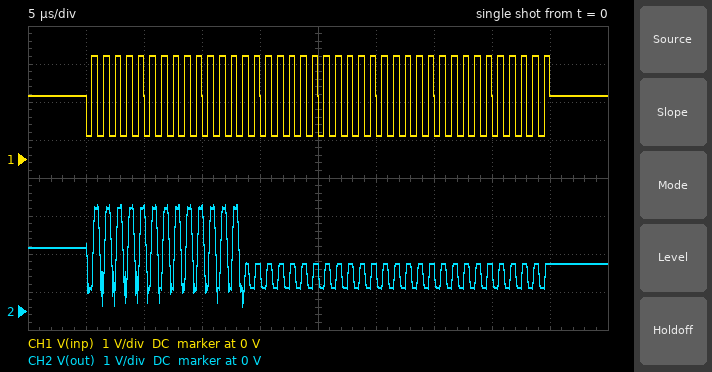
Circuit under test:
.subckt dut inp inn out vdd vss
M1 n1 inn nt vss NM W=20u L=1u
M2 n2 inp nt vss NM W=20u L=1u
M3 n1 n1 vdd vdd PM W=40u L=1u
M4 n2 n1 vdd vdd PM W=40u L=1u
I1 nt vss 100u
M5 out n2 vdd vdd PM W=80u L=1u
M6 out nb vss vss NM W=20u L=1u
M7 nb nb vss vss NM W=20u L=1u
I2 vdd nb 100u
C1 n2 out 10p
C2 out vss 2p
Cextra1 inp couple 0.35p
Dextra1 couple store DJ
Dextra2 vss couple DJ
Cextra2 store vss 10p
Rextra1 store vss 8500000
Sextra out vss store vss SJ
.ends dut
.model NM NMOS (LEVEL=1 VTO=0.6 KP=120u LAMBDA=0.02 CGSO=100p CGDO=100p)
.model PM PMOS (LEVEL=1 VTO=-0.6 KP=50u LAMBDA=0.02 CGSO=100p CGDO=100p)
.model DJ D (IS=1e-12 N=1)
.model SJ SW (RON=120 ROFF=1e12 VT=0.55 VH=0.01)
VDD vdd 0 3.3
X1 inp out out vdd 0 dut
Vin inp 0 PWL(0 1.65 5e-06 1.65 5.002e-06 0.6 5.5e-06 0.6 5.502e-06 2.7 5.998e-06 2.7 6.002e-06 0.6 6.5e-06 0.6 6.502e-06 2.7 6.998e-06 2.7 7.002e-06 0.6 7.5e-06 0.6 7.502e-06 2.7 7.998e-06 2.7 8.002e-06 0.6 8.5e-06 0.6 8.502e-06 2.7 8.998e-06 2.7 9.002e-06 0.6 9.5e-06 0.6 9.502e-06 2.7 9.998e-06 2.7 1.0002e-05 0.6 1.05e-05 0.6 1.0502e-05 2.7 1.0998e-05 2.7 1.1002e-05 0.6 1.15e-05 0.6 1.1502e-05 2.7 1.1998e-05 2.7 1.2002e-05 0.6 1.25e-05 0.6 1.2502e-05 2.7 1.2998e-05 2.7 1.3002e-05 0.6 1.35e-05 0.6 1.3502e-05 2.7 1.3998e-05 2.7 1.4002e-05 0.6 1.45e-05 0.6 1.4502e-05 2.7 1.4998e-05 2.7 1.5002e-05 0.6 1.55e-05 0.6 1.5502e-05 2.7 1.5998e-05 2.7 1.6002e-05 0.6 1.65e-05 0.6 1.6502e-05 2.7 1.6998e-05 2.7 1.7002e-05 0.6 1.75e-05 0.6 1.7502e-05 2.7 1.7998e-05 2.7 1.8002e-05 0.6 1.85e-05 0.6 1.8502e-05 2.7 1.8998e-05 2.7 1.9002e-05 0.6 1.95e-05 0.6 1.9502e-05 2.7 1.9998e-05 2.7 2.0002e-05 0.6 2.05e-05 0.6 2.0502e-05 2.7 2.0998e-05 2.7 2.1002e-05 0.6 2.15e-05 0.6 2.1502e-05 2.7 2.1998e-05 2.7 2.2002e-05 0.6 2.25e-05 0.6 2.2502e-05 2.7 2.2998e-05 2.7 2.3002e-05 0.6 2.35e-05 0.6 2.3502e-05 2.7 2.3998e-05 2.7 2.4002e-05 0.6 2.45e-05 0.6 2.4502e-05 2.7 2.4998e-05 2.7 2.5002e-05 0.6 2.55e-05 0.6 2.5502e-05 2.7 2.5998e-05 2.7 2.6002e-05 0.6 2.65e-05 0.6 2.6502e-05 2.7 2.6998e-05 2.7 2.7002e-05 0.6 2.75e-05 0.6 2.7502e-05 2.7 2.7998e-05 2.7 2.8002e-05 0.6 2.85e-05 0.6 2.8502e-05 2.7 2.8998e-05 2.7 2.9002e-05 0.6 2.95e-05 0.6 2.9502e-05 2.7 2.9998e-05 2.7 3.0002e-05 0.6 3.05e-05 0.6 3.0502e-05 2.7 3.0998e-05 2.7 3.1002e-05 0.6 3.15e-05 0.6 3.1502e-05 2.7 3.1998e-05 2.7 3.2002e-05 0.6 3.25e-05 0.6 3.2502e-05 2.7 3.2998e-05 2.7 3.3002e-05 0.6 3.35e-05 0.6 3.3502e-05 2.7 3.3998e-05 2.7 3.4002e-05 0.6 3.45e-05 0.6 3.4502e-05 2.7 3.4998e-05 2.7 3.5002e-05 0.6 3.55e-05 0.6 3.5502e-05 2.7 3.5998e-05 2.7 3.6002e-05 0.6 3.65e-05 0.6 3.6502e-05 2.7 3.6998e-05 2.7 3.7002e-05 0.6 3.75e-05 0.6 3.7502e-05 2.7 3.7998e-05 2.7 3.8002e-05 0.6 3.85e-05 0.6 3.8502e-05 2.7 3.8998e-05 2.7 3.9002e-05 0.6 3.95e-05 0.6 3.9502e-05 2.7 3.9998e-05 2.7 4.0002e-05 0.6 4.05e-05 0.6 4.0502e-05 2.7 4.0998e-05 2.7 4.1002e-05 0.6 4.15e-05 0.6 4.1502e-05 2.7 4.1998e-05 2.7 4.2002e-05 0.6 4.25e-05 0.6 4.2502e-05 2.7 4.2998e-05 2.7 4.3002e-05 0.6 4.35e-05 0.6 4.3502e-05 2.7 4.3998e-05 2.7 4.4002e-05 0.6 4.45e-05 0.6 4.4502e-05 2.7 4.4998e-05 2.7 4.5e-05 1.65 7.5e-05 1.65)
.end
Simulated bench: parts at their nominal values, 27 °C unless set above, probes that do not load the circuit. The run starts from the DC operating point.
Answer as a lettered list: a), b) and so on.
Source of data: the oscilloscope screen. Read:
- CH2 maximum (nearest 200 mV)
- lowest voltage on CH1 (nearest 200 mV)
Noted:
a) 2.8 V
b) 600 mV
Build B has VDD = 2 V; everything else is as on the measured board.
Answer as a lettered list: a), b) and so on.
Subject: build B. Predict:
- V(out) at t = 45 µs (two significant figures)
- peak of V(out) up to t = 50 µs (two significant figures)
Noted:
a) 600 mV
b) 2.0 V
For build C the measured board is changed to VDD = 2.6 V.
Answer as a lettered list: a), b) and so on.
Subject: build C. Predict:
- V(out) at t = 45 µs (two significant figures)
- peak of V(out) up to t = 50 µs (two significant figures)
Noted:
a) 880 mV
b) 2.6 V
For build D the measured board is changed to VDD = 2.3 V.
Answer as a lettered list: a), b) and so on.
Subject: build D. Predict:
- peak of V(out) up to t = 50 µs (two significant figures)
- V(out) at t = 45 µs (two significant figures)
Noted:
a) 2.3 V
b) 740 mV
